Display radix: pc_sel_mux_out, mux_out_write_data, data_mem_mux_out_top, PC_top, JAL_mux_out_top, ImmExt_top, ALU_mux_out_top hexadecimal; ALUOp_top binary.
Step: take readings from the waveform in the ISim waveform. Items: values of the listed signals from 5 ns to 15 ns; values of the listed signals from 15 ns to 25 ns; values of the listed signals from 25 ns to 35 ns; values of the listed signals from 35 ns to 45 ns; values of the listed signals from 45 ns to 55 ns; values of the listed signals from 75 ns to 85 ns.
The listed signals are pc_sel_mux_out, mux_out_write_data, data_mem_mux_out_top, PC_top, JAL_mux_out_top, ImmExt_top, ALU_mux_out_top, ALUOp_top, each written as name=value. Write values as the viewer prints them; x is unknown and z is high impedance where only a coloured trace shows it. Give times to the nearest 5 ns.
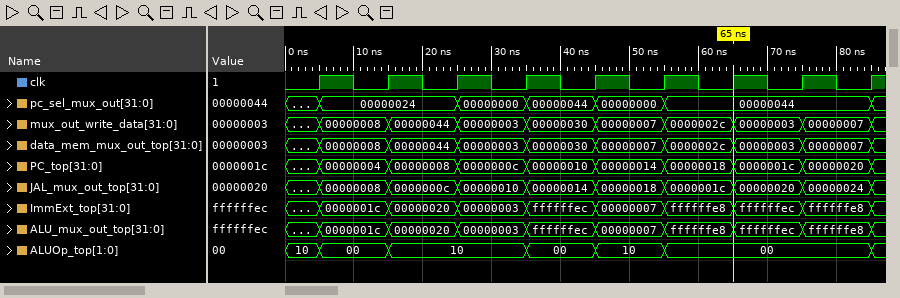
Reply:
pc_sel_mux_out=00000024, mux_out_write_data=00000008, data_mem_mux_out_top=00000008, PC_top=00000004, JAL_mux_out_top=00000008, ImmExt_top=0000001c, ALU_mux_out_top=0000001c, ALUOp_top=00
pc_sel_mux_out=00000024, mux_out_write_data=00000044, data_mem_mux_out_top=00000044, PC_top=00000008, JAL_mux_out_top=0000000c, ImmExt_top=00000020, ALU_mux_out_top=00000020, ALUOp_top=10
pc_sel_mux_out=00000000, mux_out_write_data=00000003, data_mem_mux_out_top=00000003, PC_top=0000000c, JAL_mux_out_top=00000010, ImmExt_top=00000003, ALU_mux_out_top=00000003, ALUOp_top=10
pc_sel_mux_out=00000044, mux_out_write_data=00000030, data_mem_mux_out_top=00000030, PC_top=00000010, JAL_mux_out_top=00000014, ImmExt_top=ffffffec, ALU_mux_out_top=ffffffec, ALUOp_top=00
pc_sel_mux_out=00000000, mux_out_write_data=00000007, data_mem_mux_out_top=00000007, PC_top=00000014, JAL_mux_out_top=00000018, ImmExt_top=00000007, ALU_mux_out_top=00000007, ALUOp_top=10
pc_sel_mux_out=00000044, mux_out_write_data=00000007, data_mem_mux_out_top=00000007, PC_top=00000020, JAL_mux_out_top=00000024, ImmExt_top=ffffffe8, ALU_mux_out_top=ffffffe8, ALUOp_top=00
